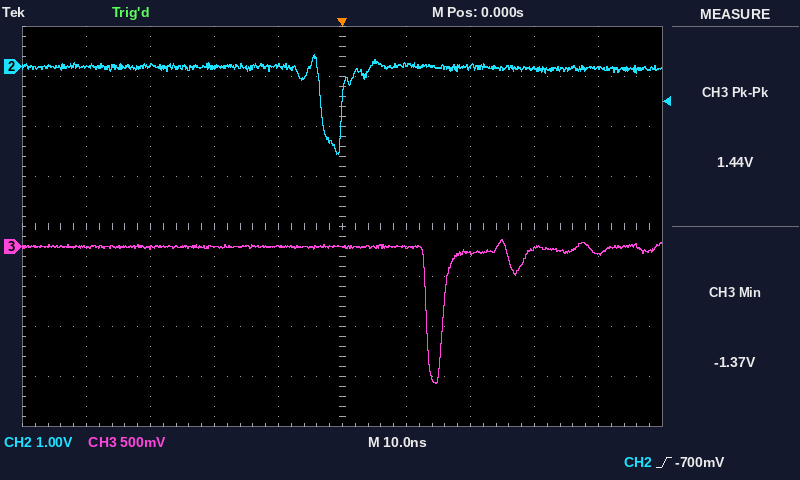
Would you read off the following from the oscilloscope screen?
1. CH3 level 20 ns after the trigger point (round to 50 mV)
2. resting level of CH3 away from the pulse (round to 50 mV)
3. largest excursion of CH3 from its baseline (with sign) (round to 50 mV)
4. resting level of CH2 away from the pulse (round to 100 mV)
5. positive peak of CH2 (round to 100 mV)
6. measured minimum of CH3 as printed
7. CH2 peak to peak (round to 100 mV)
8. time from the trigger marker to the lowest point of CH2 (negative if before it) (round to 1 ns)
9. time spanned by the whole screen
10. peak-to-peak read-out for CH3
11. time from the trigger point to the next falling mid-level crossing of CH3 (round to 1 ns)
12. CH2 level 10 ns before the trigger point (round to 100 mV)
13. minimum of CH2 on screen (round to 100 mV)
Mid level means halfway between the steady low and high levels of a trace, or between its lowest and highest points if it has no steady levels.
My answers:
-50 mV
0 mV
-1.35 V
0.0 V
200 mV
-1.37 V
2.0 V
-1 ns
100 ns
1.44 V
13 ns
0.0 V
-1.8 V
